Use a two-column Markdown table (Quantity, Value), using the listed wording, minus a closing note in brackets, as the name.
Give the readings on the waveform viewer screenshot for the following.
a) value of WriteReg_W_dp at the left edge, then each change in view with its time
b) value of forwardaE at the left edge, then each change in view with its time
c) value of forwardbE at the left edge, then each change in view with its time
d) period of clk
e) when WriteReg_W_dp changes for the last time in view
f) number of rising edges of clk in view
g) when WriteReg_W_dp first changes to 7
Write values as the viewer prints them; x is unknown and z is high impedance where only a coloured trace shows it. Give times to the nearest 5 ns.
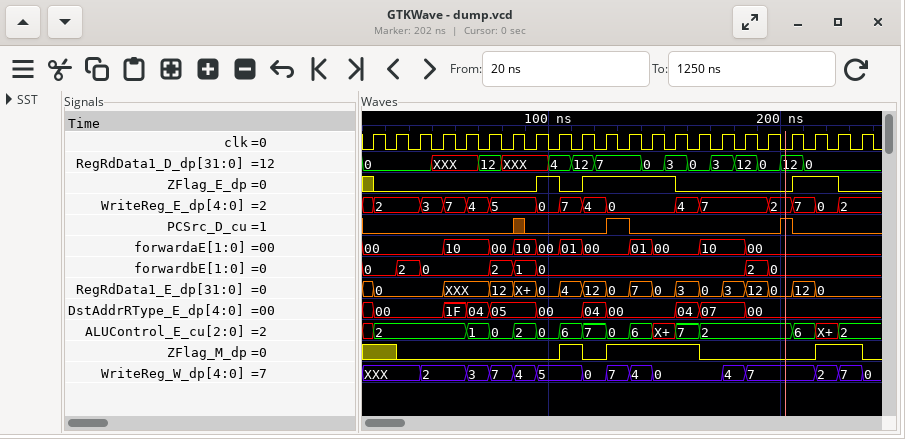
| Quantity | Value |
|---|---|
| value of WriteReg_W_dp at the left edge, then each change in view with its time | XXX, 2 at 45 ns, 3 at 65 ns, 7 at 75 ns, 4 at 85 ns, 5 at 95 ns, 0 at 115 ns, 7 at 125 ns, 4 at 135 ns, 0 at 145 ns, 4 at 175 ns, 7 at 185 ns, 2 at 215 ns, 7 at 225 ns, 0 at 235 ns |
| value of forwardaE at the left edge, then each change in view with its time | 00, 10 at 55 ns, 00 at 75 ns, 10 at 85 ns, 00 at 95 ns, 01 at 105 ns, 00 at 115 ns, 01 at 135 ns, 00 at 145 ns, 10 at 165 ns, 00 at 185 ns |
| value of forwardbE at the left edge, then each change in view with its time | 0, 2 at 35 ns, 0 at 45 ns, 2 at 75 ns, 1 at 85 ns, 0 at 95 ns, 2 at 185 ns, 0 at 195 ns |
| period of clk | 10 ns |
| when WriteReg_W_dp changes for the last time in view | 235 ns |
| number of rising edges of clk in view | 22 |
| when WriteReg_W_dp first changes to 7 | 75 ns |
